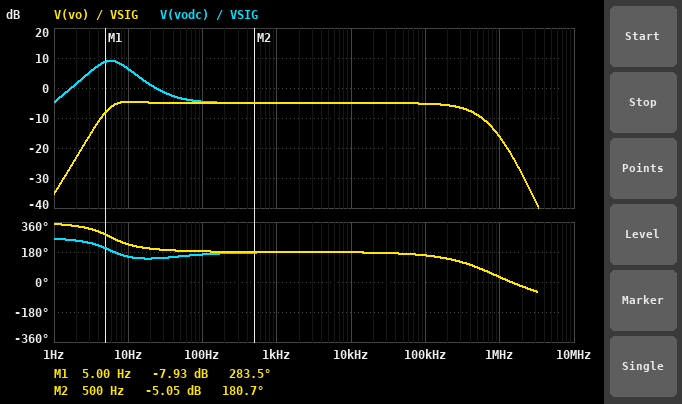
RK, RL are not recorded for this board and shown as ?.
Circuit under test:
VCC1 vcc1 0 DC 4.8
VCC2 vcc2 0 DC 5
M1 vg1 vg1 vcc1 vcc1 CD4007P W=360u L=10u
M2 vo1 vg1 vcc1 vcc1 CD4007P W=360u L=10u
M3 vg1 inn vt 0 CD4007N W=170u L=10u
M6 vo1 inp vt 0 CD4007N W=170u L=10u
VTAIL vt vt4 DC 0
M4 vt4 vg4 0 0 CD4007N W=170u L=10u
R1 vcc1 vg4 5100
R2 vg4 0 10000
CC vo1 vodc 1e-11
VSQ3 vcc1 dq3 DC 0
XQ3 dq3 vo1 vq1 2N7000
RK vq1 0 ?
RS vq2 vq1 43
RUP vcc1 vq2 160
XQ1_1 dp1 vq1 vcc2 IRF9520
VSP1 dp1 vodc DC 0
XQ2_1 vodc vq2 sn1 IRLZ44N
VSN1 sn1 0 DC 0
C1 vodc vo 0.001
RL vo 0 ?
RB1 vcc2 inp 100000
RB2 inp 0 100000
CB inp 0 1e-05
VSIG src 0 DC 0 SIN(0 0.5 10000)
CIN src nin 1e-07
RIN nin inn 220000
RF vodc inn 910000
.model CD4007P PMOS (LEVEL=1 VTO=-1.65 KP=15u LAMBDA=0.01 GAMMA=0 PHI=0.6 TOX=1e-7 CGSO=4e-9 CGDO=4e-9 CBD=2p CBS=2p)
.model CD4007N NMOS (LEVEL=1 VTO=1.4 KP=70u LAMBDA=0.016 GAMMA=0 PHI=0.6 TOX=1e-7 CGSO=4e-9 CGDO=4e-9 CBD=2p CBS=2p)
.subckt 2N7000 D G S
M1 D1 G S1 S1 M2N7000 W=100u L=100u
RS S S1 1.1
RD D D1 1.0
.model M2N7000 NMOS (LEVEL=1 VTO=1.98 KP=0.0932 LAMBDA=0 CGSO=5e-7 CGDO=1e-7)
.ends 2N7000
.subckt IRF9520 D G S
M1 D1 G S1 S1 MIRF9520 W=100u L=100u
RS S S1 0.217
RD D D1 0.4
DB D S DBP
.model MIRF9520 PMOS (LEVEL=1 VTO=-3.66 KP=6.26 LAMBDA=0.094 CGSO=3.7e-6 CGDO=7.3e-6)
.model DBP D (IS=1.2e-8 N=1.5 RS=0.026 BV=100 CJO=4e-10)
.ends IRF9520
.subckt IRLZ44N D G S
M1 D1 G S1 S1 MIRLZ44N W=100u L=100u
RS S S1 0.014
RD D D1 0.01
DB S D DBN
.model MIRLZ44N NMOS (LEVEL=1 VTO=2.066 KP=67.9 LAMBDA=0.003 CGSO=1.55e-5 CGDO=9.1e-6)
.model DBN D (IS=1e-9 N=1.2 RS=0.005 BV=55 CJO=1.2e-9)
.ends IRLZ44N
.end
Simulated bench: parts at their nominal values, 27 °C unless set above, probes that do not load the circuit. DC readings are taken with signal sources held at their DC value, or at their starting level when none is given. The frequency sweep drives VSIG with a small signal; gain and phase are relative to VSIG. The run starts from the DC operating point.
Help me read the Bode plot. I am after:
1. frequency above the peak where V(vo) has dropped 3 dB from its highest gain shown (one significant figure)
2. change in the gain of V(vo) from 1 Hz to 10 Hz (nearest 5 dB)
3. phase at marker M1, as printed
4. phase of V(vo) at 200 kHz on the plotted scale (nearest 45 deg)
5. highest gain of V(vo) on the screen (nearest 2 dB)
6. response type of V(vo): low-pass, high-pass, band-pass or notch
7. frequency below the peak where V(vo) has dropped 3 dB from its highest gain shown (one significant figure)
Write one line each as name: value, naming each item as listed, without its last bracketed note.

frequency above the peak where V(vo) has dropped 3 dB from its highest gain shown: 400 kHz
change in the gain of V(vo) from 1 Hz to 10 Hz: 30 dB
phase at marker M1, as printed: 283.5 deg
phase of V(vo) at 200 kHz on the plotted scale: 135 deg
highest gain of V(vo) on the screen: -4 dB
response type of V(vo): low-pass, high-pass, band-pass or notch: band-pass
frequency below the peak where V(vo) has dropped 3 dB from its highest gain shown: 5 Hz
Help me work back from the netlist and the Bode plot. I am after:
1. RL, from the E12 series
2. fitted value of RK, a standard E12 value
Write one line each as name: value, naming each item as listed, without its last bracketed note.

RL, from the E12 series: 4.7 Ω
fitted value of RK, a standard E12 value: 27 Ω
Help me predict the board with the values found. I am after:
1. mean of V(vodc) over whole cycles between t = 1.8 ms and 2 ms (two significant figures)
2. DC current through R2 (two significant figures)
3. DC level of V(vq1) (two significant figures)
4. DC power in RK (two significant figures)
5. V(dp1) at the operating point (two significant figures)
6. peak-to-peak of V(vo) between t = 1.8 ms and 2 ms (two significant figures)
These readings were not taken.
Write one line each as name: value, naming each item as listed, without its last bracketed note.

mean of V(vodc) over whole cycles between t = 1.8 ms and 2 ms: 2.6 V
DC current through R2: 320 µA
DC level of V(vq1): 1.3 V
DC power in RK: 66 mW
V(dp1) at the operating point: 2.6 V
peak-to-peak of V(vo) between t = 1.8 ms and 2 ms: 2.8 V
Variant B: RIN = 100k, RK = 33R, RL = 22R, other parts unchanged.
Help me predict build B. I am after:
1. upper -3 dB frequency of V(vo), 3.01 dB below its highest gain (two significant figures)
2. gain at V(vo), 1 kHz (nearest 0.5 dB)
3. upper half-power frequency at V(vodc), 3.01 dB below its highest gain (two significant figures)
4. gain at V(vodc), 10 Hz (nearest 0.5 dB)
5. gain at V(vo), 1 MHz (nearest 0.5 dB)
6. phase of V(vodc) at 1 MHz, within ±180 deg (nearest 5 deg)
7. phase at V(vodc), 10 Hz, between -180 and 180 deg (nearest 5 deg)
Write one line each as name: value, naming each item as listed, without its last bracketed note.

upper -3 dB frequency of V(vo), 3.01 dB below its highest gain: 600 kHz
gain at V(vo), 1 kHz: 11.0 dB
upper half-power frequency at V(vodc), 3.01 dB below its highest gain: 540 kHz
gain at V(vodc), 10 Hz: 11.5 dB
gain at V(vo), 1 MHz: 0.5 dB
phase of V(vodc) at 1 MHz, within ±180 deg: 10 deg
phase at V(vodc), 10 Hz, between -180 and 180 deg: -155 deg
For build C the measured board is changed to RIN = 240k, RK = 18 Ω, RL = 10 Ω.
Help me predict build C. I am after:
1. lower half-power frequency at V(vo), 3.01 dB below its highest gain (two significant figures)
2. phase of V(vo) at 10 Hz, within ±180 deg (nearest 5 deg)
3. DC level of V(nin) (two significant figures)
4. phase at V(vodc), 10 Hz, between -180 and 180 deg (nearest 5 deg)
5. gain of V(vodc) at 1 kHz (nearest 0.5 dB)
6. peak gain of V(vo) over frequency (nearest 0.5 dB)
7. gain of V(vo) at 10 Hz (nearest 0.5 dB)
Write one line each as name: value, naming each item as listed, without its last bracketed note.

lower half-power frequency at V(vo), 3.01 dB below its highest gain: 3.0 Hz
phase of V(vo) at 10 Hz, within ±180 deg: -155 deg
DC level of V(nin): 2.9 V
phase at V(vodc), 10 Hz, between -180 and 180 deg: 145 deg
gain of V(vodc) at 1 kHz: -7.5 dB
peak gain of V(vo) over frequency: -6.5 dB
gain of V(vo) at 10 Hz: -7.0 dB
